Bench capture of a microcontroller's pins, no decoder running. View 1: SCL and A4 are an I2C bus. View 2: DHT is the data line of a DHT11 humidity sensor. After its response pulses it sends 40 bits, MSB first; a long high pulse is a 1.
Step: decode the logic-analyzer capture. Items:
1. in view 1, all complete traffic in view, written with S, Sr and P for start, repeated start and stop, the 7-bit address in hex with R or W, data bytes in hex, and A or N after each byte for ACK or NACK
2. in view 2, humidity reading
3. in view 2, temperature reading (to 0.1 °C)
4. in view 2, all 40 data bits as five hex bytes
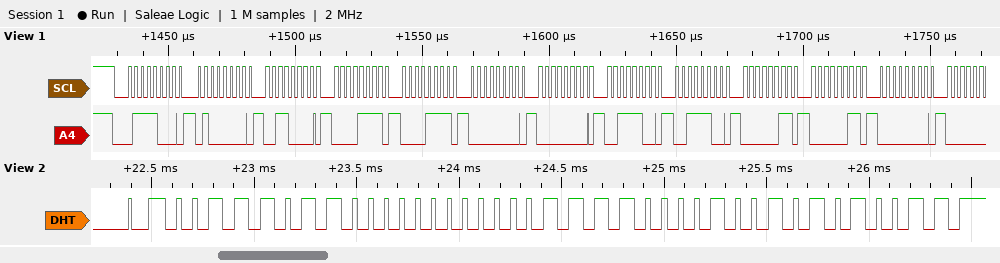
S 3CW A 40 A 30 A 0F A 0F A 00 A 00 A 3C A 3C A 03 A 03 A 00 A
59 %
15.9 °C
3B 00 0F 09 53
